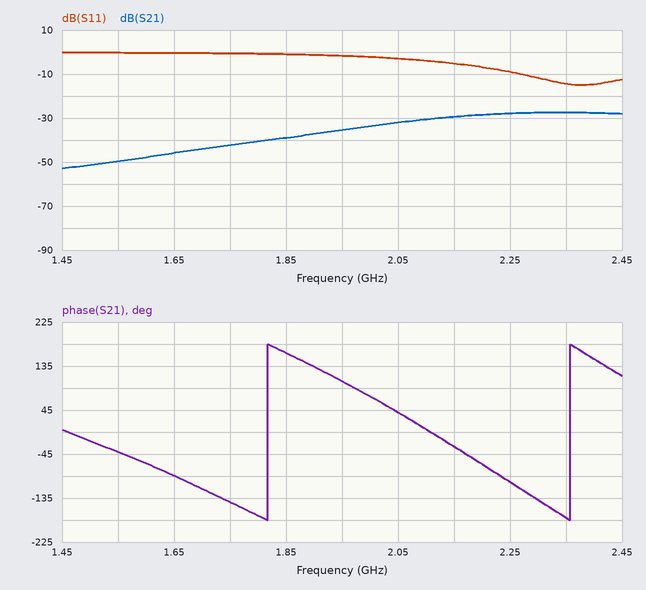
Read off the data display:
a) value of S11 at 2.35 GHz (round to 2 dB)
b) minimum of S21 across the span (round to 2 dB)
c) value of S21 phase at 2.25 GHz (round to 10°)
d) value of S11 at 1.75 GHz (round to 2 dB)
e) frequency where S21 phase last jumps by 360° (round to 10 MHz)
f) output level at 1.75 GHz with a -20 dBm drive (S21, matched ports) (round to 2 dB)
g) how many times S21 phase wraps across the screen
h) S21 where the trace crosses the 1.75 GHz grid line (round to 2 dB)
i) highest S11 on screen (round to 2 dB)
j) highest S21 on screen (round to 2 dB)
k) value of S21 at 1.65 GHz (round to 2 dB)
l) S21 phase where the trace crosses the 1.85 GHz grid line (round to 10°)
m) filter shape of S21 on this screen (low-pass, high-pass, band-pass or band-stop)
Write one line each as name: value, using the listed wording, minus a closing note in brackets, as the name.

value of S11 at 2.35 GHz: -14 dB
minimum of S21 across the span: -52 dB
value of S21 phase at 2.25 GHz: -100°
value of S11 at 1.75 GHz: 0 dB
frequency where S21 phase last jumps by 360°: 2.36 GHz
output level at 1.75 GHz with a -20 dBm drive (S21, matched ports): -62 dBm
how many times S21 phase wraps across the screen: 2
S21 where the trace crosses the 1.75 GHz grid line: -42 dB
highest S11 on screen: 0 dB
highest S21 on screen: -28 dB
value of S21 at 1.65 GHz: -46 dB
S21 phase where the trace crosses the 1.85 GHz grid line: 160°
filter shape of S21 on this screen: high-pass
